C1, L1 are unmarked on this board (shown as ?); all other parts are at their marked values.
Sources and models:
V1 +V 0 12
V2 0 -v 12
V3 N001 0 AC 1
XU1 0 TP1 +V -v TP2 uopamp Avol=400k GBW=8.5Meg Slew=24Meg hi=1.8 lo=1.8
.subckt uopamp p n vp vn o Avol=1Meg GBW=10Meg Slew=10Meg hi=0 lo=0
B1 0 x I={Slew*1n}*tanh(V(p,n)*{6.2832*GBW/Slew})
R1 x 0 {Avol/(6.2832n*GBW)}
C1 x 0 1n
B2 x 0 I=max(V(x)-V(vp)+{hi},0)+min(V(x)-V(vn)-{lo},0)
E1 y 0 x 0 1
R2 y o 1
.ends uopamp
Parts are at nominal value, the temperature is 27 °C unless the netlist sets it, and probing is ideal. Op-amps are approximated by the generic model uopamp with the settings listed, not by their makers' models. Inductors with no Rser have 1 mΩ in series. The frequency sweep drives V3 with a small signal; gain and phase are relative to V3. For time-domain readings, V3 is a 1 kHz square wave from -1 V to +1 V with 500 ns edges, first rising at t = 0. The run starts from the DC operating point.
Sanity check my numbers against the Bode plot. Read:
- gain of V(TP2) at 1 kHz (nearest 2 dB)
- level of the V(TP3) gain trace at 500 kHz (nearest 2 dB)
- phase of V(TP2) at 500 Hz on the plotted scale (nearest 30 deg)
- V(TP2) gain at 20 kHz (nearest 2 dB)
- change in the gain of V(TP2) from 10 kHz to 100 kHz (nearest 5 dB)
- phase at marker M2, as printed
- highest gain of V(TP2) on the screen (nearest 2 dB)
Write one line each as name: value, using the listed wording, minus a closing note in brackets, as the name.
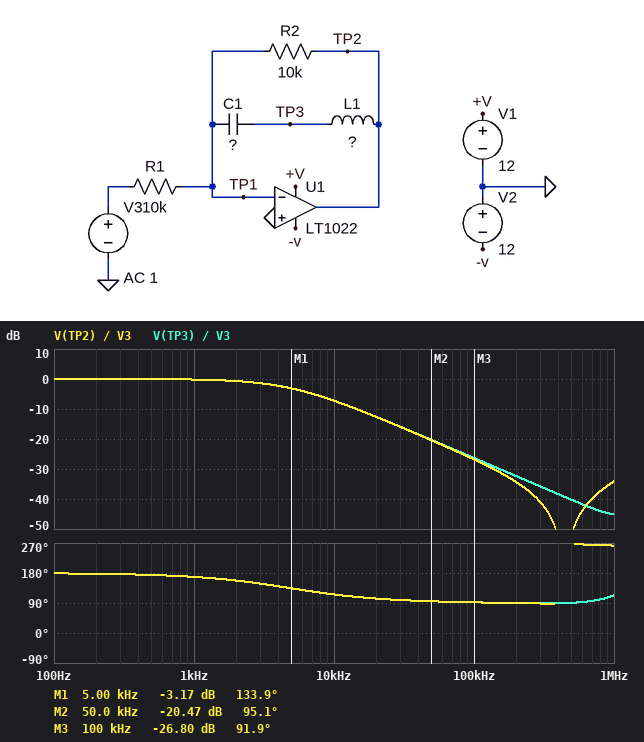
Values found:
gain of V(TP2) at 1 kHz: 0 dB
level of the V(TP3) gain trace at 500 kHz: -40 dB
phase of V(TP2) at 500 Hz on the plotted scale: 180 deg
V(TP2) gain at 20 kHz: -12 dB
change in the gain of V(TP2) from 10 kHz to 100 kHz: -20 dB
phase at marker M2, as printed: 95.1 deg
highest gain of V(TP2) on the screen: 0 dB
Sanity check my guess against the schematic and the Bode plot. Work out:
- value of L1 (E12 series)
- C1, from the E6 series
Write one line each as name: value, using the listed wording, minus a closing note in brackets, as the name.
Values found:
value of L1: 39 µH
C1, from the E6 series: 3.3 nF
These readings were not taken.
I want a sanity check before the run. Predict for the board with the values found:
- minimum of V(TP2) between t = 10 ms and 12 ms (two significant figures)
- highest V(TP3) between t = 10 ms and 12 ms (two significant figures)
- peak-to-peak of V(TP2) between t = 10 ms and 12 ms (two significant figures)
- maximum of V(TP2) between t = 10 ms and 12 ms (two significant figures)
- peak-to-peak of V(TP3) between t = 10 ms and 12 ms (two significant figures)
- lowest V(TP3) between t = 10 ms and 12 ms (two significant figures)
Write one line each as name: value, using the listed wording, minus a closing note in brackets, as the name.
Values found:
minimum of V(TP2) between t = 10 ms and 12 ms: -1.0 V
highest V(TP3) between t = 10 ms and 12 ms: 1.0 V
peak-to-peak of V(TP2) between t = 10 ms and 12 ms: 2.0 V
maximum of V(TP2) between t = 10 ms and 12 ms: 1.0 V
peak-to-peak of V(TP3) between t = 10 ms and 12 ms: 2.0 V
lowest V(TP3) between t = 10 ms and 12 ms: -1.0 V
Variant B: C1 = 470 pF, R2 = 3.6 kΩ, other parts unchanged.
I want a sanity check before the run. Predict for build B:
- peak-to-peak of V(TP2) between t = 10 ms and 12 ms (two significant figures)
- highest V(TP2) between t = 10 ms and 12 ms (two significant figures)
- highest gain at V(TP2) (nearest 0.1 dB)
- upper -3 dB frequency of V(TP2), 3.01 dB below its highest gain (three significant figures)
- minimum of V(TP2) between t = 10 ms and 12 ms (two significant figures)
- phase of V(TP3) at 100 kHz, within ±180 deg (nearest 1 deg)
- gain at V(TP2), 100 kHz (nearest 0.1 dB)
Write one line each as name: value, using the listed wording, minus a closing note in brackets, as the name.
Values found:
peak-to-peak of V(TP2) between t = 10 ms and 12 ms: 720 mV
highest V(TP2) between t = 10 ms and 12 ms: 360 mV
highest gain at V(TP2): -8.9 dB
upper -3 dB frequency of V(TP2), 3.01 dB below its highest gain: 93.1 kHz
minimum of V(TP2) between t = 10 ms and 12 ms: -360 mV
phase of V(TP3) at 100 kHz, within ±180 deg: 132 deg
gain at V(TP2), 100 kHz: -12.2 dB
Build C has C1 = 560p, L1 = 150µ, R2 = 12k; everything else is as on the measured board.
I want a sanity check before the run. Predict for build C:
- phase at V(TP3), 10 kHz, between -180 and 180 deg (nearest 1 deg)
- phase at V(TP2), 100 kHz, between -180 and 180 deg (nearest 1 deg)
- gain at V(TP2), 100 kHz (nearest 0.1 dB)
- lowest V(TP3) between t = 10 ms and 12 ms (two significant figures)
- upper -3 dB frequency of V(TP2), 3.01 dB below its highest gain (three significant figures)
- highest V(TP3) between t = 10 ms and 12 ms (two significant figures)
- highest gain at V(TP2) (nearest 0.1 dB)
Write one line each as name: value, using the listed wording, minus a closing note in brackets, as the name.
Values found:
phase at V(TP3), 10 kHz, between -180 and 180 deg: 157 deg
phase at V(TP2), 100 kHz, between -180 and 180 deg: 102 deg
gain at V(TP2), 100 kHz: -11.5 dB
lowest V(TP3) between t = 10 ms and 12 ms: -1.2 V
upper -3 dB frequency of V(TP2), 3.01 dB below its highest gain: 23.6 kHz
highest V(TP3) between t = 10 ms and 12 ms: 1.2 V
highest gain at V(TP2): 1.6 dB
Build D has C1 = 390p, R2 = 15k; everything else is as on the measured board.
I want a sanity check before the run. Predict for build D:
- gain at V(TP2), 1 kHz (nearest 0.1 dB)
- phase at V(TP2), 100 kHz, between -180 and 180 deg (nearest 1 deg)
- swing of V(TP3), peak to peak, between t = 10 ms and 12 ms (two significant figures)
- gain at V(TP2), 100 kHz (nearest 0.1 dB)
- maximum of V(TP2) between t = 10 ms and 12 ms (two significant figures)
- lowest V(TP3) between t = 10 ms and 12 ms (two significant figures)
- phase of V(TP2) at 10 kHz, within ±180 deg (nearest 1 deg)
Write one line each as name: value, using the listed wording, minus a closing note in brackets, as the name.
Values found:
gain at V(TP2), 1 kHz: 3.5 dB
phase at V(TP2), 100 kHz, between -180 and 180 deg: 104 deg
swing of V(TP3), peak to peak, between t = 10 ms and 12 ms: 3.0 V
gain at V(TP2), 100 kHz: -8.2 dB
maximum of V(TP2) between t = 10 ms and 12 ms: 1.5 V
lowest V(TP3) between t = 10 ms and 12 ms: -1.5 V
phase of V(TP2) at 10 kHz, within ±180 deg: 160 deg
